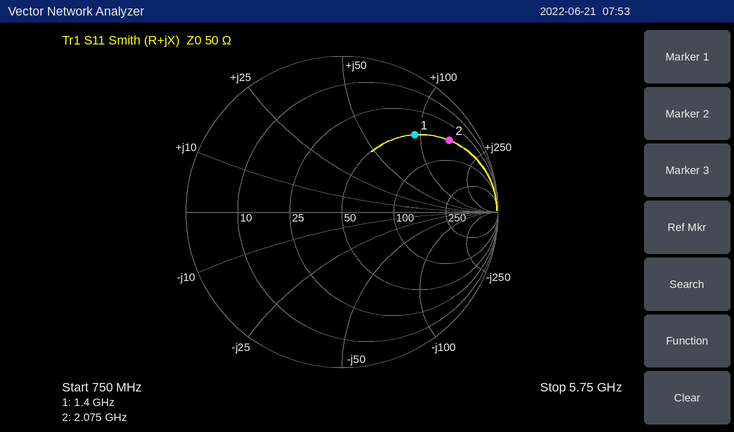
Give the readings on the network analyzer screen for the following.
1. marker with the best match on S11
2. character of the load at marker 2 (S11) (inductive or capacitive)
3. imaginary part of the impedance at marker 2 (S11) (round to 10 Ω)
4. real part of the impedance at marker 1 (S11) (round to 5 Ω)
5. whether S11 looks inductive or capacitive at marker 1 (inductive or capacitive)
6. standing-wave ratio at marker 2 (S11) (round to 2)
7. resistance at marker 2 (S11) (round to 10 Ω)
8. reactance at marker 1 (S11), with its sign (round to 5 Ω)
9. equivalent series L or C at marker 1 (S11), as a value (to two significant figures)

marker 1
inductive
+150 Ω
50 Ω
inductive
10
50 Ω
+95 Ω
11 nH
